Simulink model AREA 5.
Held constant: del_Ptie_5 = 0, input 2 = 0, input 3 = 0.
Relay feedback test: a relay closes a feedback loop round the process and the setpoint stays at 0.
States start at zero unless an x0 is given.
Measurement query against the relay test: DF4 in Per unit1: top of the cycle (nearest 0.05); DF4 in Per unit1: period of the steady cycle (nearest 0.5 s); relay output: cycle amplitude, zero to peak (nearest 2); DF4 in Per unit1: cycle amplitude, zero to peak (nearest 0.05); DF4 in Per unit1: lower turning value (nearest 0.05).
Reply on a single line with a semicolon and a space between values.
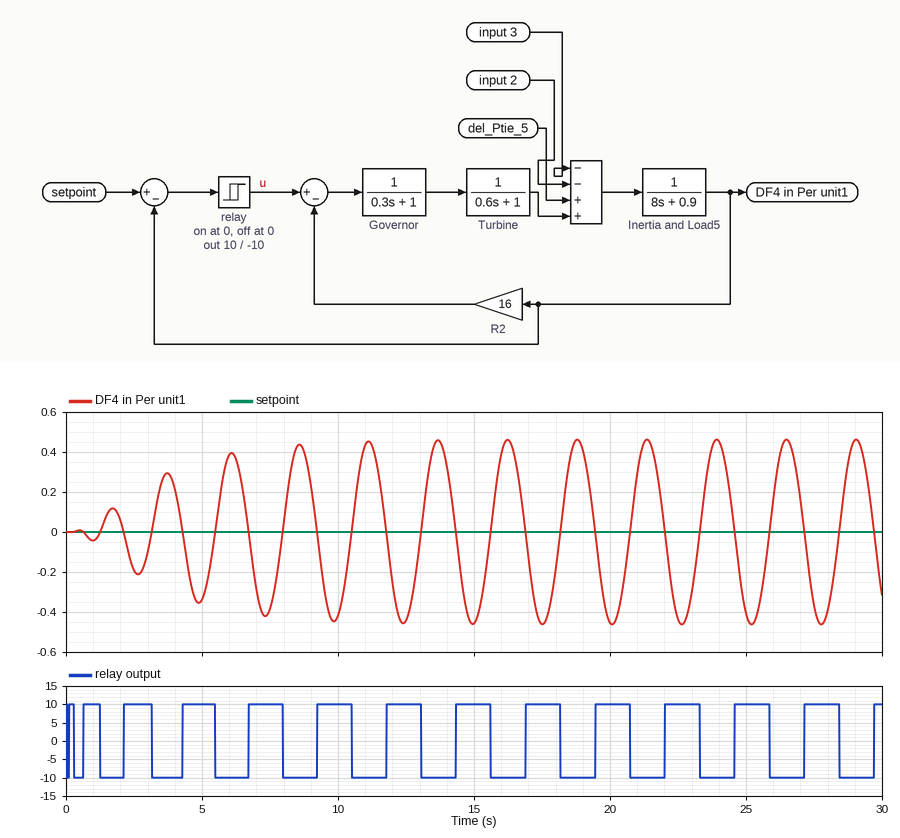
0.45; 2.5 s; 10; 0.45; -0.45
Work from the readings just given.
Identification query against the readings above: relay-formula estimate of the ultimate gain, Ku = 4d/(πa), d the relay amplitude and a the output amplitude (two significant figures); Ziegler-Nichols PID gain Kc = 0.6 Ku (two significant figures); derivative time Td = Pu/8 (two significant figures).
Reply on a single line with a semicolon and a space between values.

28; 17; 0.31 s
